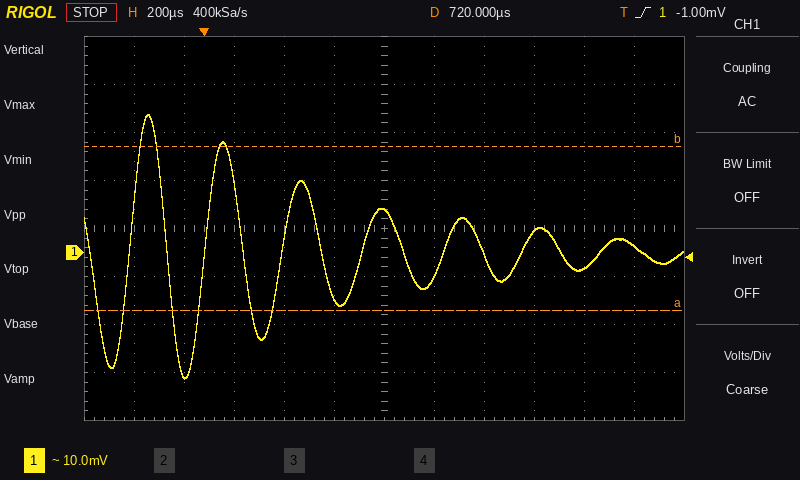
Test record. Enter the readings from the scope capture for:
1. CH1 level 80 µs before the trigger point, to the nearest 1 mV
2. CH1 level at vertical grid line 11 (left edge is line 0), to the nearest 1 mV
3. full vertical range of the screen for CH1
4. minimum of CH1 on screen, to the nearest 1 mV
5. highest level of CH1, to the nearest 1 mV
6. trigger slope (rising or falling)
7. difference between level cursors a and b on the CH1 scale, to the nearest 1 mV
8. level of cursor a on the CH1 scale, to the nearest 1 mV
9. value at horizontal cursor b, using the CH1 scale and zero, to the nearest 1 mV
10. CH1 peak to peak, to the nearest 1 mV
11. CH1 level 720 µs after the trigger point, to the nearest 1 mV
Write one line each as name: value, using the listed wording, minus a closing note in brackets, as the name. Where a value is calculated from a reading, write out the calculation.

CH1 level 80 µs before the trigger point, to the nearest 1 mV: -25 mV
CH1 level at vertical grid line 11 (left edge is line 0), to the nearest 1 mV: 1 mV
full vertical range of the screen for CH1: 80 mV
minimum of CH1 on screen, to the nearest 1 mV: -26 mV
highest level of CH1, to the nearest 1 mV: 29 mV
trigger slope: rising
difference between level cursors a and b on the CH1 scale, to the nearest 1 mV: 34 mV
level of cursor a on the CH1 scale, to the nearest 1 mV: -12 mV
value at horizontal cursor b, using the CH1 scale and zero, to the nearest 1 mV: 22 mV
CH1 peak to peak, to the nearest 1 mV: 29 mV − (-26 mV) = 55 mV
CH1 level 720 µs after the trigger point, to the nearest 1 mV: 9 mV
